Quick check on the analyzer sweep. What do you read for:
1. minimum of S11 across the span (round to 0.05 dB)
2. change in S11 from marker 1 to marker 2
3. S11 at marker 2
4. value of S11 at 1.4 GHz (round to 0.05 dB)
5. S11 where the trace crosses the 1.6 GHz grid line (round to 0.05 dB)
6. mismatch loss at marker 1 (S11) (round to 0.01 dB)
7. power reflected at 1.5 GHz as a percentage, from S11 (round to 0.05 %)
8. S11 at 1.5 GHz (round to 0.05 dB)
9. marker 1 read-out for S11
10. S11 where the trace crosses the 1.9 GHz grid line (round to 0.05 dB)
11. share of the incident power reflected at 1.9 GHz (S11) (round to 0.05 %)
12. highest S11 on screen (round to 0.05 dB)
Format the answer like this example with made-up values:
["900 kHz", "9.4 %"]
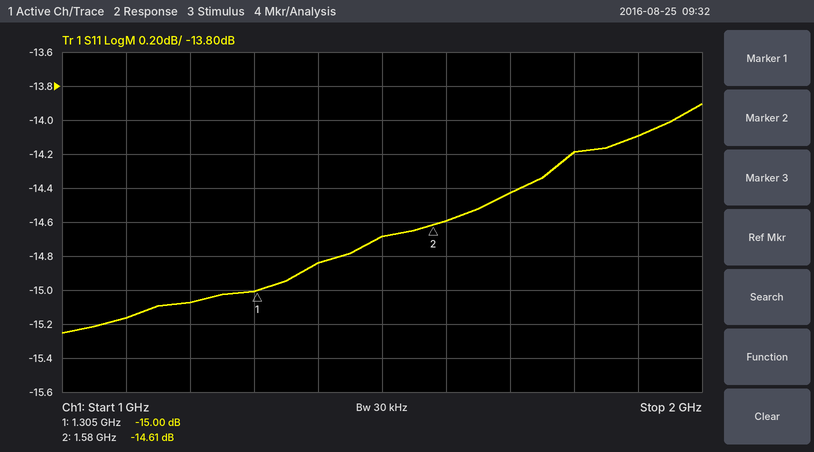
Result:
["-15.25 dB", "0.39 dB", "-14.61 dB", "-14.85 dB", "-14.60 dB", "0.14 dB", "3.40 %", "-14.70 dB", "-15.00 dB", "-14.10 dB", "3.90 %", "-13.90 dB"]
